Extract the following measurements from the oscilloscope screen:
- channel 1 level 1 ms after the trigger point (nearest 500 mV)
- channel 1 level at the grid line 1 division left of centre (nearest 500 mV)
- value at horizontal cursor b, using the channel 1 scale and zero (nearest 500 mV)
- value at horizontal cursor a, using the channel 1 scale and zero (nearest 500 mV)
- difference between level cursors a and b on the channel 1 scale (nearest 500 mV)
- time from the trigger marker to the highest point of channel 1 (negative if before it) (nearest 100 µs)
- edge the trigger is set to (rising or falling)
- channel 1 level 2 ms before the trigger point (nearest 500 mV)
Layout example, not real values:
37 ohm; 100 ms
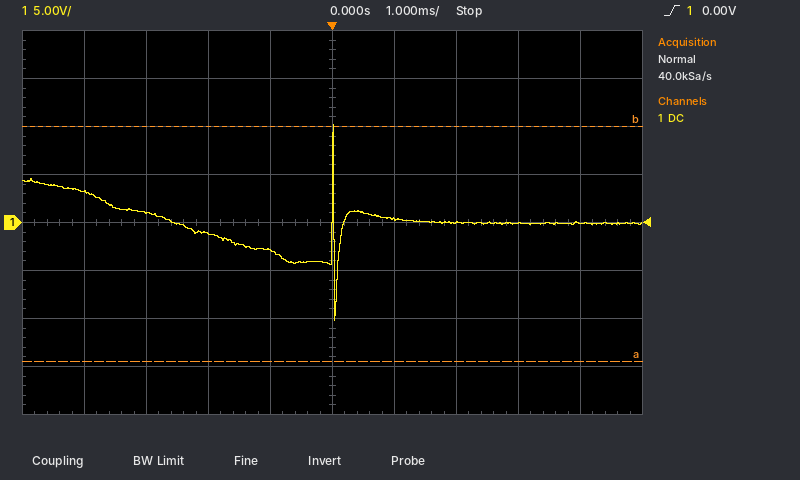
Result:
500 mV; -3.0 V; 10.0 V; -14.5 V; 24.5 V; 0.0 ms; rising; -1.0 V
